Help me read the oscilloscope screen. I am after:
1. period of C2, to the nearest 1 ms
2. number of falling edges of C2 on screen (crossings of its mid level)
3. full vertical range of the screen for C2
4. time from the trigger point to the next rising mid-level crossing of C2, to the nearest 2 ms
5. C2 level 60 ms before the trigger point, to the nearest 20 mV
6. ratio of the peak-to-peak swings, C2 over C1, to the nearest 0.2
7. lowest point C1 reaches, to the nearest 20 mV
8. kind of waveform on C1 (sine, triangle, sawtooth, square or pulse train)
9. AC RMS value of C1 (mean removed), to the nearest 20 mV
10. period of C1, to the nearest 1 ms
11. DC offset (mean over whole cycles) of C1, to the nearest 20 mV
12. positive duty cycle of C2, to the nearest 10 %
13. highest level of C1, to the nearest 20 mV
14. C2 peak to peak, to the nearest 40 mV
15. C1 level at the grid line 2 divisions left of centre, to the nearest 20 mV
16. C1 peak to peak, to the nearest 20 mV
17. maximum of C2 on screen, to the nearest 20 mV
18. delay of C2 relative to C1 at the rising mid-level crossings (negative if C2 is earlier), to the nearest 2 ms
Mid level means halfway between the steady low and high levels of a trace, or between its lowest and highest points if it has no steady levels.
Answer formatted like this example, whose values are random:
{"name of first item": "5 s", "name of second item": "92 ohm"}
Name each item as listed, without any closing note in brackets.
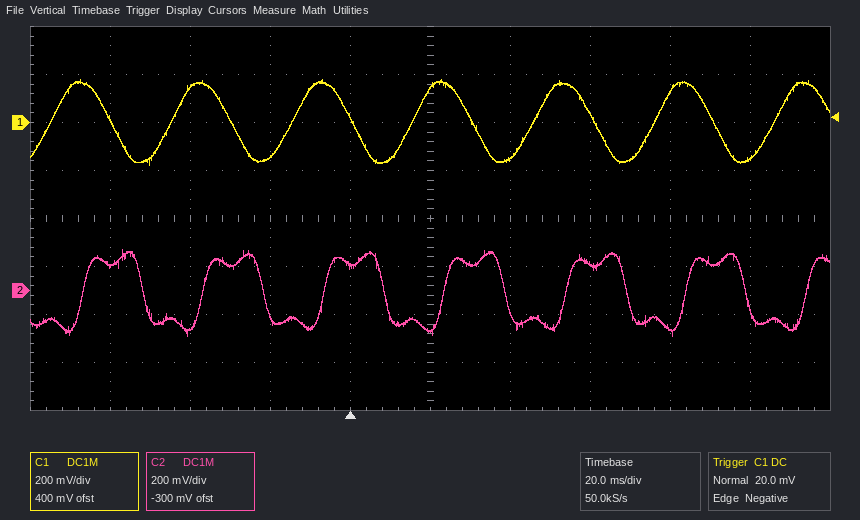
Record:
{"period of C2, to the nearest 1 ms": "30 ms", "number of falling edges of C2 on screen": "6", "full vertical range of the screen for C2": "1.6 V", "time from the trigger point to the next rising mid-level crossing of C2, to the nearest 2 ms": "24 ms", "C2 level 60 ms before the trigger point, to the nearest 20 mV": "100 mV", "ratio of the peak-to-peak swings, C2 over C1, to the nearest 0.2": "1.0", "lowest point C1 reaches, to the nearest 20 mV": "-180 mV", "kind of waveform on C1": "sine", "AC RMS value of C1 (mean removed), to the nearest 20 mV": "120 mV", "period of C1, to the nearest 1 ms": "30 ms", "DC offset (mean over whole cycles) of C1, to the nearest 20 mV": "0 mV", "positive duty cycle of C2, to the nearest 10 %": "50 %", "highest level of C1, to the nearest 20 mV": "180 mV", "C2 peak to peak, to the nearest 40 mV": "360 mV", "C1 level at the grid line 2 divisions left of centre, to the nearest 20 mV": "-140 mV", "C1 peak to peak, to the nearest 20 mV": "360 mV", "maximum of C2 on screen, to the nearest 20 mV": "180 mV", "delay of C2 relative to C1 at the rising mid-level crossings (negative if C2 is earlier), to the nearest 2 ms": "+8 ms"}
